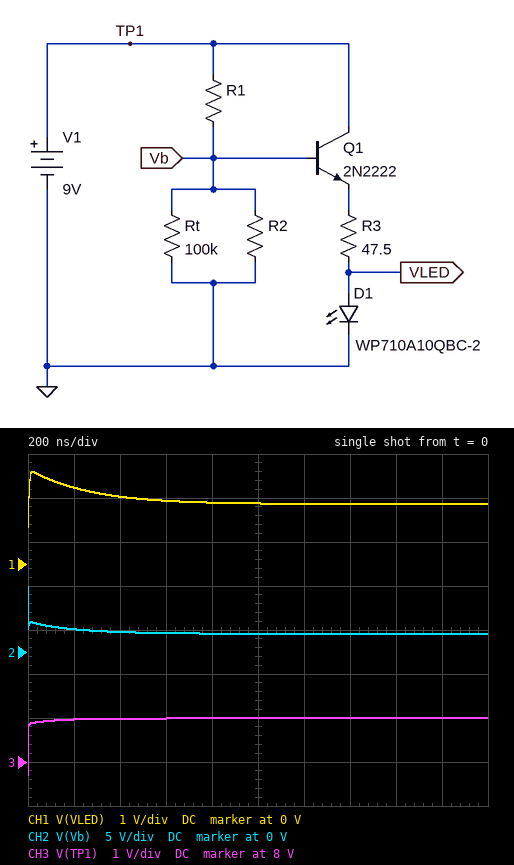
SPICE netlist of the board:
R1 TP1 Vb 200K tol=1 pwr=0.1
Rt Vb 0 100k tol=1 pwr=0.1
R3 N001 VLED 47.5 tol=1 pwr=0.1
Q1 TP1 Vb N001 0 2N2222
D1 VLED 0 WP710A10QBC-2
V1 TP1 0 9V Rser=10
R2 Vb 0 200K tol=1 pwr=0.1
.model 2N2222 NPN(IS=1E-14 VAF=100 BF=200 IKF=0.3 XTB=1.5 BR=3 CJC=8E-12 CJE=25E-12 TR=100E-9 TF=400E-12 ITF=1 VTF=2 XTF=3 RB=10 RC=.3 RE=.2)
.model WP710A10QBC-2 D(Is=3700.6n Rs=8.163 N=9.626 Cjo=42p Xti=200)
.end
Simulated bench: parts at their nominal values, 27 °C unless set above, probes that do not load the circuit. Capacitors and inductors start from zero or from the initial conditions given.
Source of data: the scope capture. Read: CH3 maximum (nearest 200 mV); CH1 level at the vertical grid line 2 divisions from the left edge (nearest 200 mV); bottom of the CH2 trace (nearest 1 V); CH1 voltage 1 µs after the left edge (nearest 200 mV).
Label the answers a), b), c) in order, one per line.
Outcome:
a) 9.0 V
b) 1.6 V
c) 2 V
d) 1.4 V
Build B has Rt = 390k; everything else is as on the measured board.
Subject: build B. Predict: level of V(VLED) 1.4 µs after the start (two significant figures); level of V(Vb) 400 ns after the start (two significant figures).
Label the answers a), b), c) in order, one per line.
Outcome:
a) 1.7 V
b) 2.6 V
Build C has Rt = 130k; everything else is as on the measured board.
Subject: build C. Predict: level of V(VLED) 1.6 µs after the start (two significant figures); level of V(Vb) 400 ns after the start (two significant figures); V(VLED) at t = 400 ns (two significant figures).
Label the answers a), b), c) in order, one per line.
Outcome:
a) 1.5 V
b) 2.4 V
c) 1.6 V
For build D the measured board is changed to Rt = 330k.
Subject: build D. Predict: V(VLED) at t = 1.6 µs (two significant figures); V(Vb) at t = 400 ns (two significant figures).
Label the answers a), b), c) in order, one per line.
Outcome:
a) 1.7 V
b) 2.6 V
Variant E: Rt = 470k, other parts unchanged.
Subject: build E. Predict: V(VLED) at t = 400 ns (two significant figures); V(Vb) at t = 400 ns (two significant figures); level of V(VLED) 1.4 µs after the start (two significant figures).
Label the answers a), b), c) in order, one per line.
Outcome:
a) 1.8 V
b) 2.6 V
c) 1.7 V
